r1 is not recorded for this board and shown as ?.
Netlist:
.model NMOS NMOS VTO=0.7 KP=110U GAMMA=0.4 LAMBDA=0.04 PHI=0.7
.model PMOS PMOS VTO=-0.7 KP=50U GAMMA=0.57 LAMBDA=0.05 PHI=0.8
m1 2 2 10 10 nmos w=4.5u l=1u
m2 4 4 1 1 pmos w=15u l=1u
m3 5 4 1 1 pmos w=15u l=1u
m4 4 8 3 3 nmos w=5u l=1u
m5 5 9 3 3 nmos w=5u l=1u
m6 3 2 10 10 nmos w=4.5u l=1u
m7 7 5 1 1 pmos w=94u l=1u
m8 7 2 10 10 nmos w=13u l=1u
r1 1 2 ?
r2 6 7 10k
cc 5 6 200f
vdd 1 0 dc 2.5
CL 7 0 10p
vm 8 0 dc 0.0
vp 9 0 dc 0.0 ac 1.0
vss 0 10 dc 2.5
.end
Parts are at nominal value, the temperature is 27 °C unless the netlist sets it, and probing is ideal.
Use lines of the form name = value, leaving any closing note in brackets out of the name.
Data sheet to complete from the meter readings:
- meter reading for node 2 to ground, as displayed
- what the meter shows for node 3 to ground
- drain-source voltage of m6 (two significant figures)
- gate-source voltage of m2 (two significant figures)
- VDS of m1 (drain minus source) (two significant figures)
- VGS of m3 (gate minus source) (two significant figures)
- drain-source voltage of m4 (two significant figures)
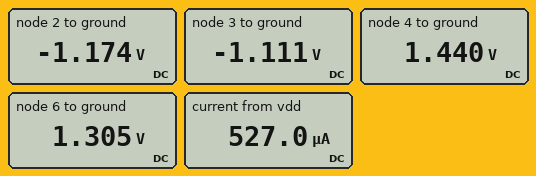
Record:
meter reading for node 2 to ground, as displayed = -1.174 V
what the meter shows for node 3 to ground = -1.111 V
drain-source voltage of m6 = 1.4 V
gate-source voltage of m2 = -1.1 V
VDS of m1 (drain minus source) = 1.3 V
VGS of m3 (gate minus source) = -1.1 V
drain-source voltage of m4 = 2.6 V
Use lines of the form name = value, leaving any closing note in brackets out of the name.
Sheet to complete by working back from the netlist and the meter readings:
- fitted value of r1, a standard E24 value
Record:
fitted value of r1, a standard E24 value = 36 kΩ
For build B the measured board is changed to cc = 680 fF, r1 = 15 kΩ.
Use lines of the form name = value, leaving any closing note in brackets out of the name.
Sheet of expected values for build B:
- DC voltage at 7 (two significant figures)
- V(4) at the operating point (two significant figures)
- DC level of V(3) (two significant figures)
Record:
DC voltage at 7 = 1.1 V
V(4) at the operating point = 1.3 V
DC level of V(3) = -1.3 V
